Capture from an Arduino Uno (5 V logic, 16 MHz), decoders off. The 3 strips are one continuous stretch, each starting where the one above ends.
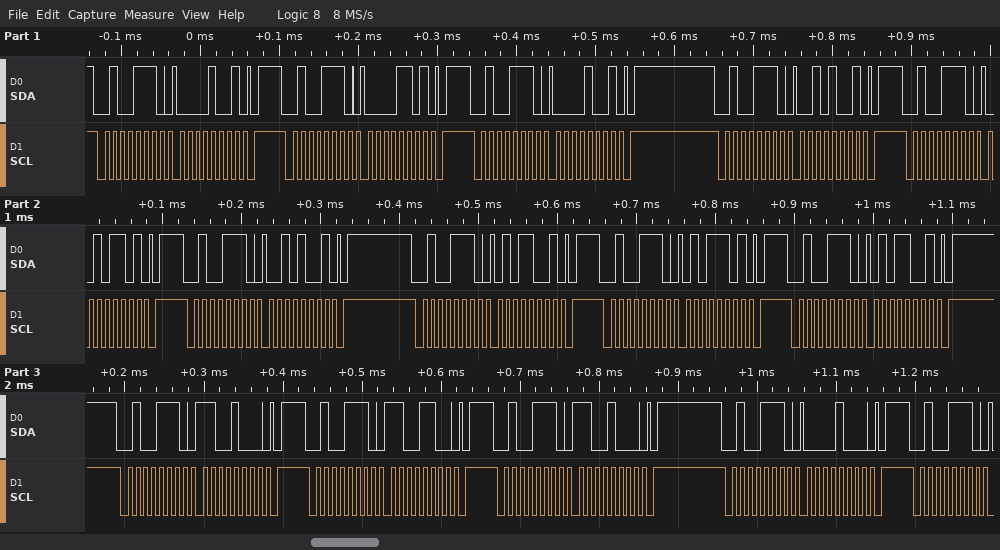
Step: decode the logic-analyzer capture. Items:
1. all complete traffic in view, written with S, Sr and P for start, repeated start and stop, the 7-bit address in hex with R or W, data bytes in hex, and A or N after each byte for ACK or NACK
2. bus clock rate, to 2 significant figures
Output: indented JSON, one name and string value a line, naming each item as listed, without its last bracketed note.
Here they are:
{
  "all complete traffic in view, written with S, Sr and P for start, repeated start and stop, the 7-bit address in hex with R or W, data bytes in hex, and A or N after each byte for ACK or NACK": "S 27W A 09 A P S 27W A 0D A P S 27W A 09 A P S 27W A 29 A P S 27W A 2D A P S 27W A 29 A P S 27W A 59 A P S 27W A 5D A P S 27W A 59 A P S 27W A C8 A P S 27W A CC A P S 27W A C8 A P S 27W A 08 A P S 27W A",
  "bus clock rate, to 2 significant figures": "100 kHz"
}
